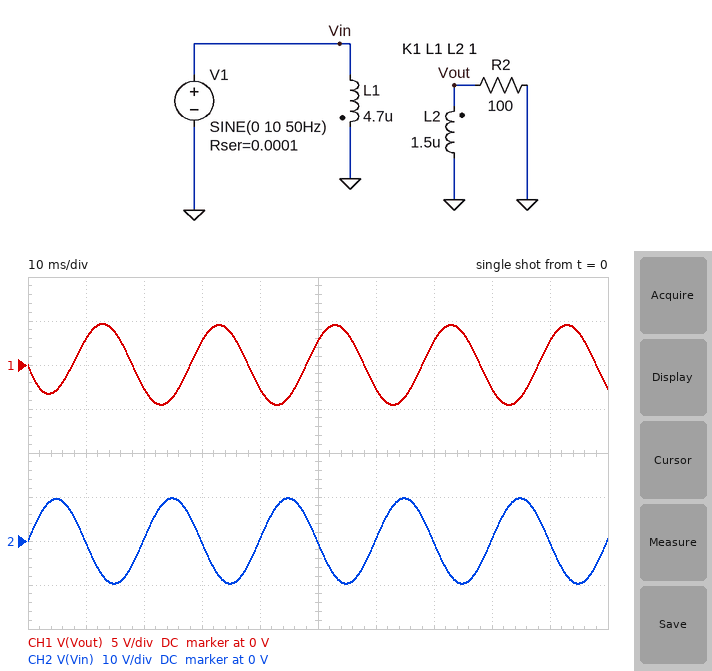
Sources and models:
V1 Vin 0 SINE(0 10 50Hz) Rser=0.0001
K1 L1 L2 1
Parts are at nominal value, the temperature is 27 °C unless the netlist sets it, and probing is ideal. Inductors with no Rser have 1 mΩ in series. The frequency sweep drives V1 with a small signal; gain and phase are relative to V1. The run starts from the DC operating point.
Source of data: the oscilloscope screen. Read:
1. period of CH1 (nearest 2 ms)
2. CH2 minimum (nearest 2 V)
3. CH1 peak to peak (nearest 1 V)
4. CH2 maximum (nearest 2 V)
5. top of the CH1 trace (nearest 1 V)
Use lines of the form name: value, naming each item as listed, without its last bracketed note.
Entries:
period of CH1: 20 ms
CH2 minimum: -10 V
CH1 peak to peak: 9 V
CH2 maximum: 10 V
top of the CH1 trace: 5 V
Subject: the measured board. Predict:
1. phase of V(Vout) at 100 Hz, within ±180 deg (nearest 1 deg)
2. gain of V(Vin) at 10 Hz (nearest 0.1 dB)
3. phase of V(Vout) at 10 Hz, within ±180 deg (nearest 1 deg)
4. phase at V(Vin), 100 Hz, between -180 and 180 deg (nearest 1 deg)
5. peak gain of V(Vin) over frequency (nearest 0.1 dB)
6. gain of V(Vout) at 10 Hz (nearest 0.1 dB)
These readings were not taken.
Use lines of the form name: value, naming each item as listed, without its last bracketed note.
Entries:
phase of V(Vout) at 100 Hz, within ±180 deg: -160 deg
gain of V(Vin) at 10 Hz: -0.8 dB
phase of V(Vout) at 10 Hz, within ±180 deg: -105 deg
phase at V(Vin), 100 Hz, between -180 and 180 deg: 2 deg
peak gain of V(Vin) over frequency: 0 dB
gain of V(Vout) at 10 Hz: -16.7 dB
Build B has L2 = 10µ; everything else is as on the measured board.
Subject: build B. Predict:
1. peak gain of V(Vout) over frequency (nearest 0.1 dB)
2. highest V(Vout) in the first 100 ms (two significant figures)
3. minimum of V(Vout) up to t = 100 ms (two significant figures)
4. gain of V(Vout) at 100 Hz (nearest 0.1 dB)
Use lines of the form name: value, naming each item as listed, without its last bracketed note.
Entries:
peak gain of V(Vout) over frequency: 3.3 dB
highest V(Vout) in the first 100 ms: 12 V
minimum of V(Vout) up to t = 100 ms: -12 V
gain of V(Vout) at 100 Hz: 2.7 dB
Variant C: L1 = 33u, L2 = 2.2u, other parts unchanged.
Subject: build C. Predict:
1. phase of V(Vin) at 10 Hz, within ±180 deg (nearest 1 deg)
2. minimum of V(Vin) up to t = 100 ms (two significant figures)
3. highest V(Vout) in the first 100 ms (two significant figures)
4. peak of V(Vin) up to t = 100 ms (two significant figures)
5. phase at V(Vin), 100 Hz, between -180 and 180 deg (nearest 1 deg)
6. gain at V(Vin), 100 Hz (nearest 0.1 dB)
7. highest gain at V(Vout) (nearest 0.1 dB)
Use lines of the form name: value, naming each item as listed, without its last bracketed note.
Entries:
phase of V(Vin) at 10 Hz, within ±180 deg: 2 deg
minimum of V(Vin) up to t = 100 ms: -10 V
highest V(Vout) in the first 100 ms: 2.7 V
peak of V(Vin) up to t = 100 ms: 10 V
phase at V(Vin), 100 Hz, between -180 and 180 deg: 0 deg
gain at V(Vin), 100 Hz: 0 dB
highest gain at V(Vout): -11.8 dB
